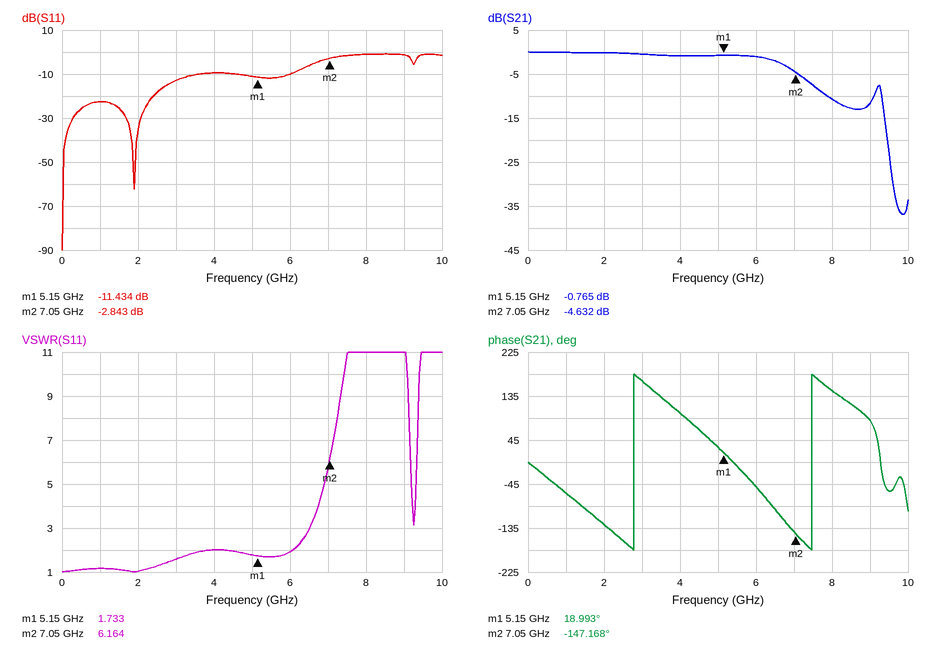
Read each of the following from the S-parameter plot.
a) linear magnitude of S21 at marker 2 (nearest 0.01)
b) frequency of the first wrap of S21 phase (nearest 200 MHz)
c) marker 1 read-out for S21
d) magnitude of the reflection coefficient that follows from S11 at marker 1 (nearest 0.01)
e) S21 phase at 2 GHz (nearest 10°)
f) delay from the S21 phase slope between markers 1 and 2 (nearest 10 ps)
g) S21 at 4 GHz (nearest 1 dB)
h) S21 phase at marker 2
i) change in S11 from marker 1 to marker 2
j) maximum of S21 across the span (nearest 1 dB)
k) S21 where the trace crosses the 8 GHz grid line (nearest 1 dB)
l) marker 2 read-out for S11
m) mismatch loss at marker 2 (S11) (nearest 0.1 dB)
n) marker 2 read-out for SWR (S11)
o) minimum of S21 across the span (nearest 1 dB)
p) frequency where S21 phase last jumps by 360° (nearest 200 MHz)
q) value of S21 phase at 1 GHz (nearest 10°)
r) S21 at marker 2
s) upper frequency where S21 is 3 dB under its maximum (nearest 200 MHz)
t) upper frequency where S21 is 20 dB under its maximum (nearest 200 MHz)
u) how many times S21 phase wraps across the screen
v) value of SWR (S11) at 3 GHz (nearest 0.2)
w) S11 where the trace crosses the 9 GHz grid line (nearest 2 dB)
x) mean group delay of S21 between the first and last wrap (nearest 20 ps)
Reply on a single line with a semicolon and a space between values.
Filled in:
0.59; 2.8 GHz; -0.765 dB; 0.27; -130°; 240 ps; -1 dB; -147.168°; 8.591 dB; 0 dB; -11 dB; -2.843 dB; 3.2 dB; 6.164; -37 dB; 7.4 GHz; -60°; -4.632 dB; 6.8 GHz; 9.4 GHz; 2; 1.6; -2 dB; 220 ps
